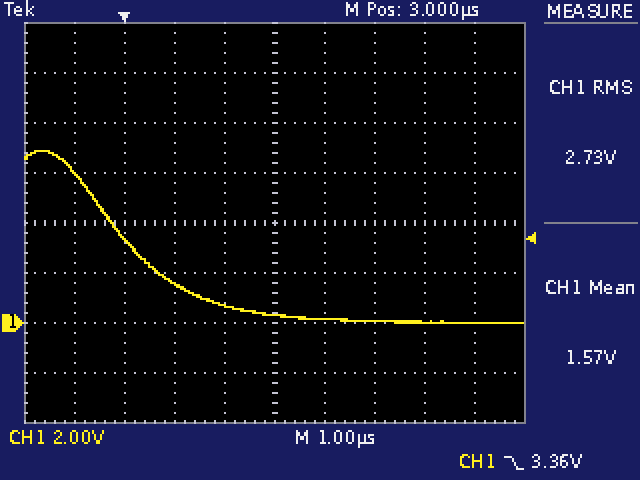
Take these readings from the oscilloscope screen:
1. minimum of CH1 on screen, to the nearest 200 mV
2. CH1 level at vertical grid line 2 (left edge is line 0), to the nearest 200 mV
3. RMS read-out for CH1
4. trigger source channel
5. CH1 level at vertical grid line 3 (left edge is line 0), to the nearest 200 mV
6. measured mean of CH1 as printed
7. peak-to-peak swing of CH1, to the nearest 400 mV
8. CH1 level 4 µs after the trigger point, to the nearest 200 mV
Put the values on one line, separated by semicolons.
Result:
0.0 V; 3.4 V; 2.73 V; CH1; 1.6 V; 1.57 V; 6.8 V; 200 mV
